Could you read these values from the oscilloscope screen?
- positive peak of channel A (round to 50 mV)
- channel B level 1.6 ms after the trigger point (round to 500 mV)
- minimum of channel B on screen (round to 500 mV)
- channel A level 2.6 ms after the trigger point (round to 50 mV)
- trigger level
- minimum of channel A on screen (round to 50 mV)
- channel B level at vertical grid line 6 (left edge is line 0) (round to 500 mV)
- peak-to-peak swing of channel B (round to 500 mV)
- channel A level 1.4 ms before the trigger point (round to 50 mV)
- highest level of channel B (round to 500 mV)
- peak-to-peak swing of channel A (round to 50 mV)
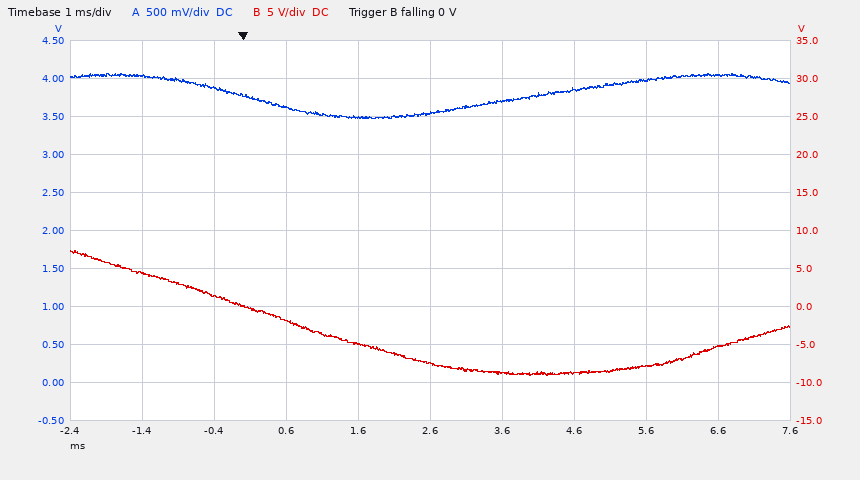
4.05 V
-5.0 V
-9.0 V
3.55 V
0 V
3.45 V
-8.5 V
16.5 V
4.05 V
7.5 V
600 mV
